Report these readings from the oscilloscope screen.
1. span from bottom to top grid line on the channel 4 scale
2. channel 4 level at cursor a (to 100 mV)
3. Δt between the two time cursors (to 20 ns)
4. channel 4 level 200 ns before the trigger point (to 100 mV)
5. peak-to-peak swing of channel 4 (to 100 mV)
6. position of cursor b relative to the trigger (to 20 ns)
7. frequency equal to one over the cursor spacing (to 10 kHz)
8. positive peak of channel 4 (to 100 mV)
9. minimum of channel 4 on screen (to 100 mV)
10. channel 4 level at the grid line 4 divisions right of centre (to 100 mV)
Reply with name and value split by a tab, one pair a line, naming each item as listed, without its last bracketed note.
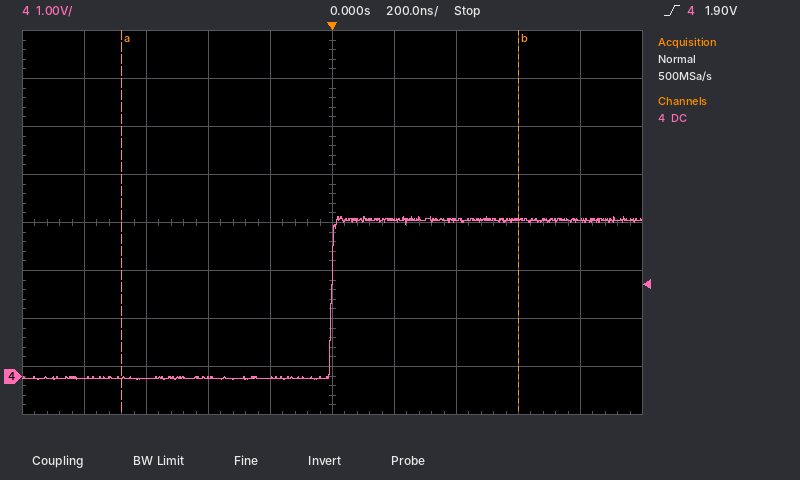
span from bottom to top grid line on the channel 4 scale	8 V
channel 4 level at cursor a	0.0 V
Δt between the two time cursors	1.28 µs
channel 4 level 200 ns before the trigger point	0.0 V
peak-to-peak swing of channel 4	3.4 V
position of cursor b relative to the trigger	+600 ns
frequency equal to one over the cursor spacing	780 kHz
positive peak of channel 4	3.3 V
minimum of channel 4 on screen	-100 mV
channel 4 level at the grid line 4 divisions right of centre	3.2 V
